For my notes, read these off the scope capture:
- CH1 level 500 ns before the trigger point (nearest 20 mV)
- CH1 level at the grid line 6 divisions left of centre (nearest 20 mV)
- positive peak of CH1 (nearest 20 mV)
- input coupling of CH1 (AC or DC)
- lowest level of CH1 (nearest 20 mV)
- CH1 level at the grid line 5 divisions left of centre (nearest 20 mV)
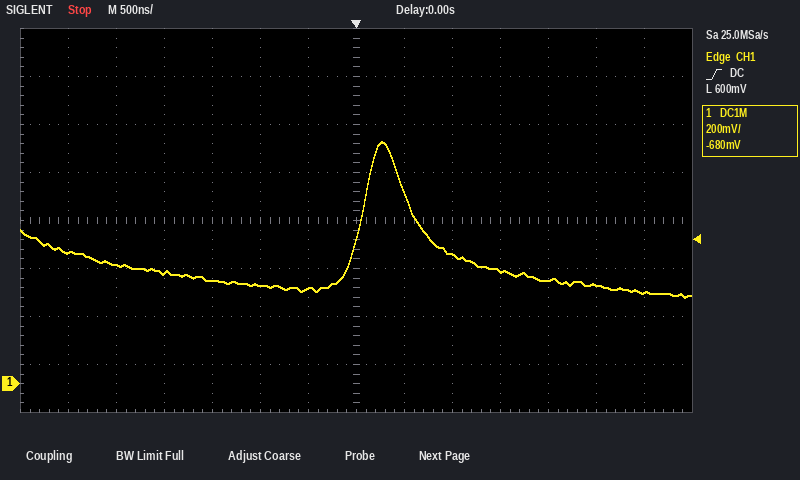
400 mV
540 mV
1.00 V
DC
360 mV
500 mV
